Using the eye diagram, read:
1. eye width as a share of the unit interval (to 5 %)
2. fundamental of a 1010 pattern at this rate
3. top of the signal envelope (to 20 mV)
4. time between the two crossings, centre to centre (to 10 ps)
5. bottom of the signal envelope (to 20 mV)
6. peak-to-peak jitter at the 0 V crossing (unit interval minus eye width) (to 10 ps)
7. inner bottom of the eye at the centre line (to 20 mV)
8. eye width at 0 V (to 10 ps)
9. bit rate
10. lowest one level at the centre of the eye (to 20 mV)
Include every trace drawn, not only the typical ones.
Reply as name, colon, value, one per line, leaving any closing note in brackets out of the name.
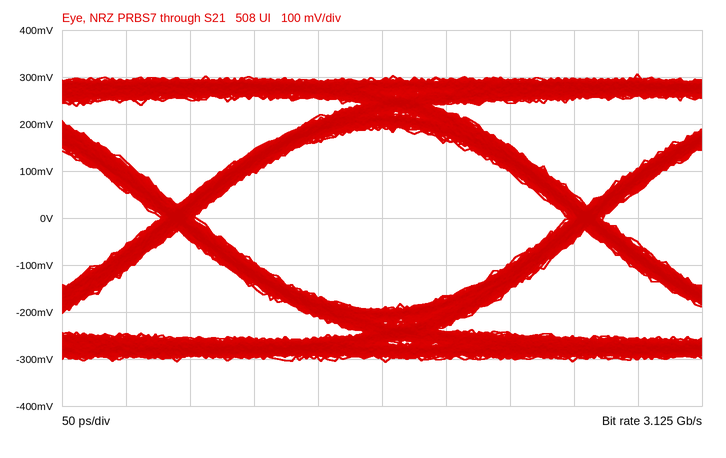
eye width as a share of the unit interval: 90 %
fundamental of a 1010 pattern at this rate: 1.5625 GHz
top of the signal envelope: 300 mV
time between the two crossings, centre to centre: 320 ps
bottom of the signal envelope: -300 mV
peak-to-peak jitter at the 0 V crossing (unit interval minus eye width): 30 ps
inner bottom of the eye at the centre line: -200 mV
eye width at 0 V: 290 ps
bit rate: 3.125 Gb/s
lowest one level at the centre of the eye: 200 mV
